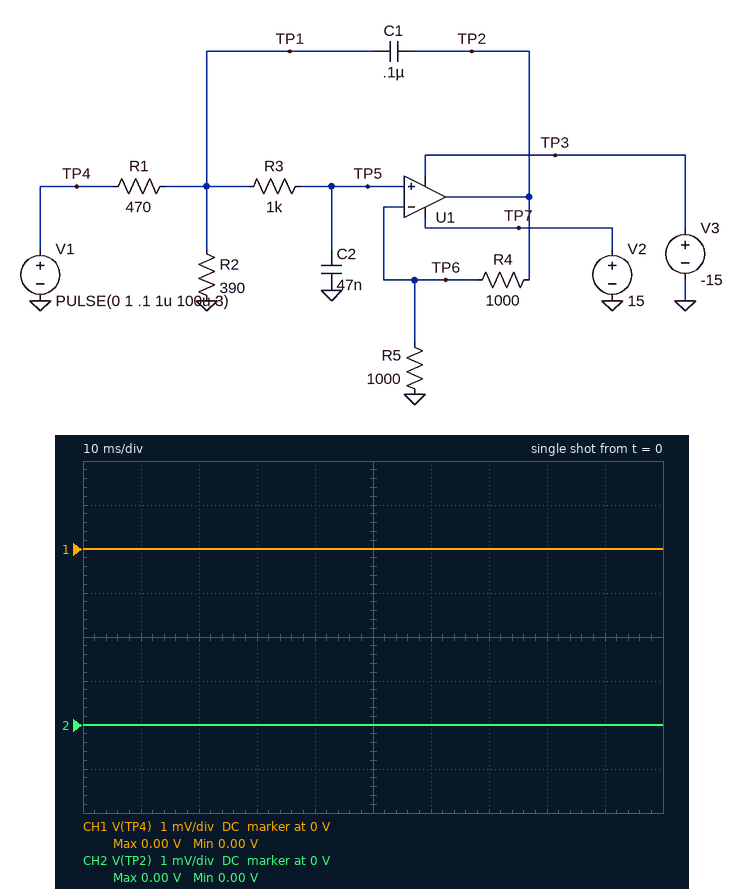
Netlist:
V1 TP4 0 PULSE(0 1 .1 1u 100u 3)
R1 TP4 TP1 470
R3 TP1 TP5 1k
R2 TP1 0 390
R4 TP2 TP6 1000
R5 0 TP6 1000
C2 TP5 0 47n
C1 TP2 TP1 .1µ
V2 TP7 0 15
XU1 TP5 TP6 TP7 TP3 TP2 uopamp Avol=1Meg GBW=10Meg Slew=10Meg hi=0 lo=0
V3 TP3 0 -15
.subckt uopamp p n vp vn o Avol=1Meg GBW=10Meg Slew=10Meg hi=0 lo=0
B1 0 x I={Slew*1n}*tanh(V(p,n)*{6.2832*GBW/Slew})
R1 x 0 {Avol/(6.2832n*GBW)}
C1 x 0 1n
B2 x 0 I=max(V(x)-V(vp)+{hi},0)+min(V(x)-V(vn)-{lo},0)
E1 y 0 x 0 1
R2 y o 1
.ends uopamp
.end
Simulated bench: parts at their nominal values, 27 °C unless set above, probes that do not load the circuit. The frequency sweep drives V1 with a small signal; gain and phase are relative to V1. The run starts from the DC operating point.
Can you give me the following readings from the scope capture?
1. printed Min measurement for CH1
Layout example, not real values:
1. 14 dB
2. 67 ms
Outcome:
1. 0.00 V
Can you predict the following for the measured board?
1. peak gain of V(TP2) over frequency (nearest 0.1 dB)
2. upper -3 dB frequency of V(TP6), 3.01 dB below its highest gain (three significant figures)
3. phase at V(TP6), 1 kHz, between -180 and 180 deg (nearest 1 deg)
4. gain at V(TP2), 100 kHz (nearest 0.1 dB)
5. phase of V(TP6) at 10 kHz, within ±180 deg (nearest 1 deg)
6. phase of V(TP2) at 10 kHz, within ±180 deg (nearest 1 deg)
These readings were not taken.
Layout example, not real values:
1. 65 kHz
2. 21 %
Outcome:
1. -0.2 dB
2. 5.72 kHz
3. -13 deg
4. -52.8 dB
5. -143 deg
6. -143 deg
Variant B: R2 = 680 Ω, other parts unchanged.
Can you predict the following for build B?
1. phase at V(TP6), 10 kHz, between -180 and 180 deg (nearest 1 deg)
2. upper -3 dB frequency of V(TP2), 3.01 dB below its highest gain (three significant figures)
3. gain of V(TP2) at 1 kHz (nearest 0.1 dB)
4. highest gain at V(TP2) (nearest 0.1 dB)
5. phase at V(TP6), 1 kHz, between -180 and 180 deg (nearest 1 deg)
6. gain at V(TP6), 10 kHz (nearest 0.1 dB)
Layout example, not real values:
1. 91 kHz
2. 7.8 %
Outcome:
1. -154 deg
2. 5.21 kHz
3. 1.7 dB
4. 3.4 dB
5. -12 deg
6. -17.9 dB
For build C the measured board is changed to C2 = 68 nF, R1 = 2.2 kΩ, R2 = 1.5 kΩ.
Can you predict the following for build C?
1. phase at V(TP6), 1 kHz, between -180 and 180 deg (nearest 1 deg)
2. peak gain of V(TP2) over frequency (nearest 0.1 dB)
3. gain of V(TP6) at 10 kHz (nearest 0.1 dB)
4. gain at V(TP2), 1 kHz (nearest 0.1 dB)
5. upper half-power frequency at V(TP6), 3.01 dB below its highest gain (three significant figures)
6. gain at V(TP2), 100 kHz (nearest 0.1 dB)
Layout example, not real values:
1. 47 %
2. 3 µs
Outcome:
1. -18 deg
2. 4.4 dB
3. -35.1 dB
4. 0.1 dB
5. 2.38 kHz
6. -69.4 dB
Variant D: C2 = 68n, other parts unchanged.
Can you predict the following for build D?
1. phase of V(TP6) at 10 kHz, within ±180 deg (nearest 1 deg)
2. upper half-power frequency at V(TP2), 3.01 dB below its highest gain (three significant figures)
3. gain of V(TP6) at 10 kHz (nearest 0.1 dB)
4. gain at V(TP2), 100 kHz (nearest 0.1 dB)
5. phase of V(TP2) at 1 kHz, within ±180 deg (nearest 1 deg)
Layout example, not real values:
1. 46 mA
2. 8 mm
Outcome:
1. -141 deg
2. 3.62 kHz
3. -22.6 dB
4. -56.0 dB
5. -22 deg
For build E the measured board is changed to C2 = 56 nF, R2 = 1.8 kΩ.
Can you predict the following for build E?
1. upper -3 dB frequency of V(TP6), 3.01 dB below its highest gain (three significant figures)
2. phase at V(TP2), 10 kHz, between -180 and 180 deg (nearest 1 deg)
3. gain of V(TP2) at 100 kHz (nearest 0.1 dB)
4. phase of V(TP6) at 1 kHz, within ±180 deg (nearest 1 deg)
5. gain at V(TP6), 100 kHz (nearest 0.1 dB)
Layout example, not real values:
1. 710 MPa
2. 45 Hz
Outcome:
1. 4.13 kHz
2. -161 deg
3. -54.3 dB
4. -15 deg
5. -60.3 dB
